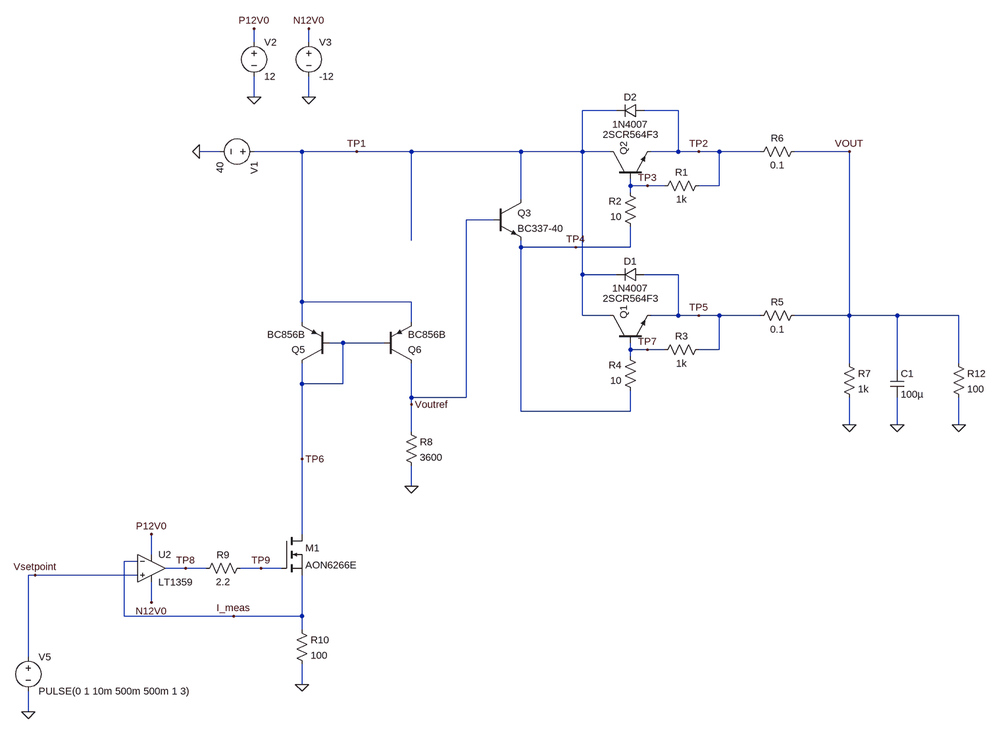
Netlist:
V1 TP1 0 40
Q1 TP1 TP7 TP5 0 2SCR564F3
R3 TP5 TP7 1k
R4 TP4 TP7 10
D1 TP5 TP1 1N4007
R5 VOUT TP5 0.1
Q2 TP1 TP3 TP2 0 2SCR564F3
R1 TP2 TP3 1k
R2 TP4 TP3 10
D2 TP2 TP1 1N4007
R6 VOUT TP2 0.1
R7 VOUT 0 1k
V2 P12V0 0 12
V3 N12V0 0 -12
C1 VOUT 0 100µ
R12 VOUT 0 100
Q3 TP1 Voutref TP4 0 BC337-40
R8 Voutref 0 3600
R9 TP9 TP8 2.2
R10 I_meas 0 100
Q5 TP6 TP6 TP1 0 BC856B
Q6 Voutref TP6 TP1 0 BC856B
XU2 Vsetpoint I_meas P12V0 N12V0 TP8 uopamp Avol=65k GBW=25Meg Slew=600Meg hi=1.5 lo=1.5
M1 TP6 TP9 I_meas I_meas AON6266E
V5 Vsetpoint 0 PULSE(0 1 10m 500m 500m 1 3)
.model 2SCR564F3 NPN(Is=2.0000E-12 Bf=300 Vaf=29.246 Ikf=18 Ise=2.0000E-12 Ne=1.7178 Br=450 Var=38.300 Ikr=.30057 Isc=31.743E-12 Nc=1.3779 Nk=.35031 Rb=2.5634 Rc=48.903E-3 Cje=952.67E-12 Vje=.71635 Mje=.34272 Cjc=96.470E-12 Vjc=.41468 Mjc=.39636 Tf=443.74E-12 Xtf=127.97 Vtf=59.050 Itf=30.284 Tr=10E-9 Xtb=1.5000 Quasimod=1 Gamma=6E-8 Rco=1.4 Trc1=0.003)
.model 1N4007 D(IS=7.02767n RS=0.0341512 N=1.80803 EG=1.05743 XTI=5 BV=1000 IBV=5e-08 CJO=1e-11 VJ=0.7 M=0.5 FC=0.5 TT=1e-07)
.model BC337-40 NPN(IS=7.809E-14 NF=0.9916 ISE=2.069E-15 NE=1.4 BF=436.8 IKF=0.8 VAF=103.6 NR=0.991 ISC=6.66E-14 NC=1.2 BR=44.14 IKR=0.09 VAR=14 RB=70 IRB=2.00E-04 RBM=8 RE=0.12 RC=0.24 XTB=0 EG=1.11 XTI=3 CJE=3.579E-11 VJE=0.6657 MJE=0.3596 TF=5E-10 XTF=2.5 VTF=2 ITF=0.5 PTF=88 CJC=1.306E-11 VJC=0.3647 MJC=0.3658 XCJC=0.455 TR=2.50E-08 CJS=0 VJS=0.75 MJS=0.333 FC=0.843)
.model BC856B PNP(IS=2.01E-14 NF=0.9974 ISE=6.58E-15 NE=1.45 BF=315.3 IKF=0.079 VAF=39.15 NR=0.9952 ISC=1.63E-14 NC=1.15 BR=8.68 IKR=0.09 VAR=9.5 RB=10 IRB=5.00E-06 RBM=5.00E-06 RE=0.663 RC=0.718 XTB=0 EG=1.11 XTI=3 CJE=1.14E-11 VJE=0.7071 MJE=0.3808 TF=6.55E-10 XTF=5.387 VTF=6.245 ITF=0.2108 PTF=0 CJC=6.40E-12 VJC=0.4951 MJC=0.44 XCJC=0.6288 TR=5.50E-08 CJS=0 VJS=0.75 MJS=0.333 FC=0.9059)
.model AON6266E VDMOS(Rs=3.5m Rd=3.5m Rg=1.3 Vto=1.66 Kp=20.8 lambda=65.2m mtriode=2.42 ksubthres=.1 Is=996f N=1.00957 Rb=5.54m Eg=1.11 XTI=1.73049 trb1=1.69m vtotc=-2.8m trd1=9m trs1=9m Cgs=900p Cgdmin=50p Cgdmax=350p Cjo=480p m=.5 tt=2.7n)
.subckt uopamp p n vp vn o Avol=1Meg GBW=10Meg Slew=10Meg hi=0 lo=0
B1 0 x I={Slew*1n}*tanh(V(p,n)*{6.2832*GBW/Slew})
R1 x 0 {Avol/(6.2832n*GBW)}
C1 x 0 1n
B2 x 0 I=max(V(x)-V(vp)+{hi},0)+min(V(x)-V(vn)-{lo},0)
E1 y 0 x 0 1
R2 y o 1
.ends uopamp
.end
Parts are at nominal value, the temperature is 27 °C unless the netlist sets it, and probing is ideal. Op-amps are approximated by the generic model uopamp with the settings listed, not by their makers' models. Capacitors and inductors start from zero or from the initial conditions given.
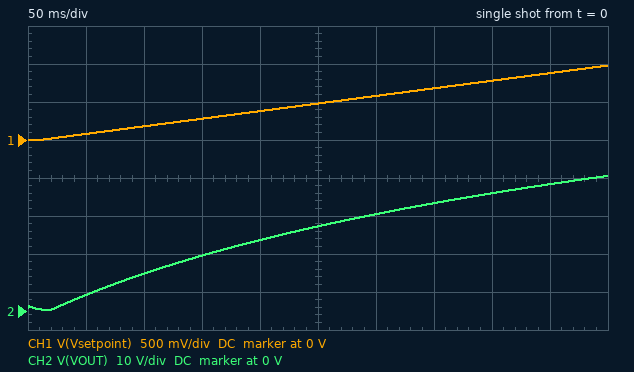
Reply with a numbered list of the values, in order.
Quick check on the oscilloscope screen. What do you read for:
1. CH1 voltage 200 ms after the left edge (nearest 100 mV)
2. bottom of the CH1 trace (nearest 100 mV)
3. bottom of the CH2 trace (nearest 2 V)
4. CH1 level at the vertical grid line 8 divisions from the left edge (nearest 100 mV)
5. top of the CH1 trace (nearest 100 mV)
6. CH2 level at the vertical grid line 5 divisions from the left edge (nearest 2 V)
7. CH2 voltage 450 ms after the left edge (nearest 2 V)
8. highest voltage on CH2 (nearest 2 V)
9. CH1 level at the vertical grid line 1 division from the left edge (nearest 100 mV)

1. 400 mV
2. 0 V
3. 0 V
4. 800 mV
5. 1.0 V
6. 22 V
7. 34 V
8. 36 V
9. 100 mV
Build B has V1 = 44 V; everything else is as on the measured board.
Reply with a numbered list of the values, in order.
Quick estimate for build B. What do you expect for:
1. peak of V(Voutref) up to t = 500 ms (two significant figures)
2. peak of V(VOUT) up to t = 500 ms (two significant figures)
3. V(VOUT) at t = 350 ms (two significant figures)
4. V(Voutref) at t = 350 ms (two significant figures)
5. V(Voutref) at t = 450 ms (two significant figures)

1. 39 V
2. 37 V
3. 30 V
4. 31 V
5. 36 V
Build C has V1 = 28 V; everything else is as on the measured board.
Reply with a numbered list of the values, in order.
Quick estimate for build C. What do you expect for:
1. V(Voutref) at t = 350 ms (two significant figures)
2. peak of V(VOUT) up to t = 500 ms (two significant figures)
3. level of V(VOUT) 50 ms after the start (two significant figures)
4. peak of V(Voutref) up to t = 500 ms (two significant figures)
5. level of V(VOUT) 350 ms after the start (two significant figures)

1. 25 V
2. 27 V
3. 3.4 V
4. 28 V
5. 24 V
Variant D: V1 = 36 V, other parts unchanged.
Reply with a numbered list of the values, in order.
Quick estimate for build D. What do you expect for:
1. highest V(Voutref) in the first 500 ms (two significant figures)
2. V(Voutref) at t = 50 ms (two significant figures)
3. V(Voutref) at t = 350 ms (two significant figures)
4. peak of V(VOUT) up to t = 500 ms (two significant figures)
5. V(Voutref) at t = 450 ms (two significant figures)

1. 35 V
2. 5.1 V
3. 28 V
4. 34 V
5. 33 V
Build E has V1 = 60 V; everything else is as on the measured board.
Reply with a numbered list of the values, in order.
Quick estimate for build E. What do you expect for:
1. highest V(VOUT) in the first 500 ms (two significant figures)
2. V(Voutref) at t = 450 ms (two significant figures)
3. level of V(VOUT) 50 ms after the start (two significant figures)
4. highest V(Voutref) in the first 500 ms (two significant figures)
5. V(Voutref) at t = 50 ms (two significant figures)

1. 44 V
2. 43 V
3. 5.6 V
4. 45 V
5. 6.8 V
